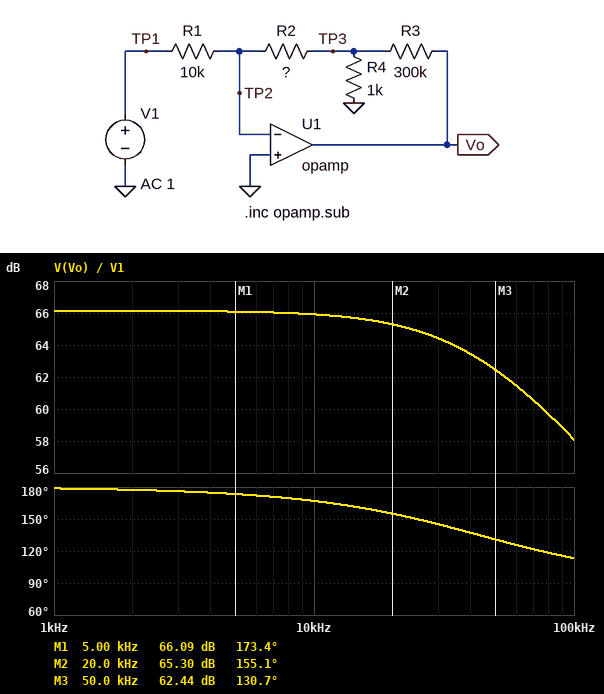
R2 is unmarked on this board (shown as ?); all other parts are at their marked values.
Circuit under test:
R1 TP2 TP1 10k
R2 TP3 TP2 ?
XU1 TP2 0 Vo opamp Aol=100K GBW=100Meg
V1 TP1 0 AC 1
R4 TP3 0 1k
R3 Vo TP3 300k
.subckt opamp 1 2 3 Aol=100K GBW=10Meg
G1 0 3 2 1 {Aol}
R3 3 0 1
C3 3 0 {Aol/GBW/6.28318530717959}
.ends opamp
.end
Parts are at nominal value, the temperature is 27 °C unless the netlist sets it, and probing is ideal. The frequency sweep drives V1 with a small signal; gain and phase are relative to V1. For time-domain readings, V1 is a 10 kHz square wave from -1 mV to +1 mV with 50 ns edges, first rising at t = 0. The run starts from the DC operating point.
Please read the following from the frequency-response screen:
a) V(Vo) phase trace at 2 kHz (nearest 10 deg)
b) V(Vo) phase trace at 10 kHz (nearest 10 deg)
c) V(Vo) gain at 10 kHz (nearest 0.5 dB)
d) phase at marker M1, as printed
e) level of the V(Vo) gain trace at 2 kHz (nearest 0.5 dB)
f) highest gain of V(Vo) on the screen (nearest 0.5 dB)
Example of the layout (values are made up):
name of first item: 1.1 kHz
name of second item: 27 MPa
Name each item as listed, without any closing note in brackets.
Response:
V(Vo) phase trace at 2 kHz: 180 deg
V(Vo) phase trace at 10 kHz: 170 deg
V(Vo) gain at 10 kHz: 66.0 dB
phase at marker M1, as printed: 173.4 deg
level of the V(Vo) gain trace at 2 kHz: 66.0 dB
highest gain of V(Vo) on the screen: 66.0 dB
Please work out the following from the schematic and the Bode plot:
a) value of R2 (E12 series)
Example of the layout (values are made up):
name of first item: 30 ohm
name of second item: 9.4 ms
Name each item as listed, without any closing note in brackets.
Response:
value of R2: 68 kΩ
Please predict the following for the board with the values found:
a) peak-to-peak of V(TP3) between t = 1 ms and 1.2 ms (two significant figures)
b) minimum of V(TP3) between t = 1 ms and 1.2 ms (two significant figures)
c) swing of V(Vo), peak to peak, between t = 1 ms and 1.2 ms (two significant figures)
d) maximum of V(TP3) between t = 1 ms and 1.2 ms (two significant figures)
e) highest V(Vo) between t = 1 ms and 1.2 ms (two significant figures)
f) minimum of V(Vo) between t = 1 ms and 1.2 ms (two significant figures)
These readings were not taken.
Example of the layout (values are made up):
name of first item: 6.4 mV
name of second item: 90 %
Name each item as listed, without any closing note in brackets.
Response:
peak-to-peak of V(TP3) between t = 1 ms and 1.2 ms: 13 mV
minimum of V(TP3) between t = 1 ms and 1.2 ms: -6.6 mV
swing of V(Vo), peak to peak, between t = 1 ms and 1.2 ms: 4.1 V
maximum of V(TP3) between t = 1 ms and 1.2 ms: 6.6 mV
highest V(Vo) between t = 1 ms and 1.2 ms: 2.0 V
minimum of V(Vo) between t = 1 ms and 1.2 ms: -2.0 V
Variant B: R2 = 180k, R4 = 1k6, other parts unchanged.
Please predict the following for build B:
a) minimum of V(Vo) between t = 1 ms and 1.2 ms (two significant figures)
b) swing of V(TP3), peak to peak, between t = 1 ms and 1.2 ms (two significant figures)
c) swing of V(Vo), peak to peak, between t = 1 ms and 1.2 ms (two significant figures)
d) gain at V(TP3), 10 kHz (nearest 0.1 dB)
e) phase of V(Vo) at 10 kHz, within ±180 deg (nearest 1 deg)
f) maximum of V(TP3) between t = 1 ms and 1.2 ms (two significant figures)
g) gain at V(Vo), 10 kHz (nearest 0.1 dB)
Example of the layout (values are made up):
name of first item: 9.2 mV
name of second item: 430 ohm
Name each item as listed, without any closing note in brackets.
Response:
minimum of V(Vo) between t = 1 ms and 1.2 ms: -3.3 V
swing of V(TP3), peak to peak, between t = 1 ms and 1.2 ms: 35 mV
swing of V(Vo), peak to peak, between t = 1 ms and 1.2 ms: 6.6 V
gain at V(TP3), 10 kHz: 24.3 dB
phase of V(Vo) at 10 kHz, within ±180 deg: 161 deg
maximum of V(TP3) between t = 1 ms and 1.2 ms: 17 mV
gain at V(Vo), 10 kHz: 69.9 dB
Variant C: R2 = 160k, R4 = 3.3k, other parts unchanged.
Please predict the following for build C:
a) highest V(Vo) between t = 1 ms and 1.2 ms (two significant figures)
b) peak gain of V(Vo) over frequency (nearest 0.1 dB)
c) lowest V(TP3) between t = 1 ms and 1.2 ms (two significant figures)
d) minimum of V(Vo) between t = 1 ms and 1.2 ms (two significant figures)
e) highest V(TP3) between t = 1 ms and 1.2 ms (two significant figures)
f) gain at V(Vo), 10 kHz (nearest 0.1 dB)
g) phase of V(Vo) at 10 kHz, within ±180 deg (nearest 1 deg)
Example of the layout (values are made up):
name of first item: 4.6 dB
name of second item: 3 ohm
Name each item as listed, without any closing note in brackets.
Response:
highest V(Vo) between t = 1 ms and 1.2 ms: 1.5 V
peak gain of V(Vo) over frequency: 63.4 dB
lowest V(TP3) between t = 1 ms and 1.2 ms: -16 mV
minimum of V(Vo) between t = 1 ms and 1.2 ms: -1.5 V
highest V(TP3) between t = 1 ms and 1.2 ms: 16 mV
gain at V(Vo), 10 kHz: 63.3 dB
phase of V(Vo) at 10 kHz, within ±180 deg: 171 deg
